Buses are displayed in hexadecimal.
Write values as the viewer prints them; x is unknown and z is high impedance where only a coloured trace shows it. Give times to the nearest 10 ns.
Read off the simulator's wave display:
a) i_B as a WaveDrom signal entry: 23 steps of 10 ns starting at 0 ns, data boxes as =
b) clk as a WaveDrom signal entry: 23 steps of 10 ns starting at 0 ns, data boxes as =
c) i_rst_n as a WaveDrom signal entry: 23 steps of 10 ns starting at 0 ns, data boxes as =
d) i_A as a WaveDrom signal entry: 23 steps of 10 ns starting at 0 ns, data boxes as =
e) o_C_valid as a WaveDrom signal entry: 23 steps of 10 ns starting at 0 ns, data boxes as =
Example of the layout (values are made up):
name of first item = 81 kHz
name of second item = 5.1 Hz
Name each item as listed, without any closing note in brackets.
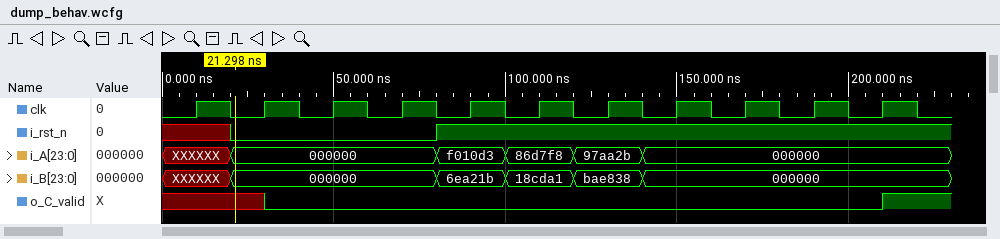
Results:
i_B as a WaveDrom signal entry: 23 steps of 10 ns starting at 0 ns, data boxes as = = {name: 'i_B', wave: 'x.=.....=.=.=.=........', data: '000000 6ea21b 18cda1 bae838 000000'}
clk as a WaveDrom signal entry: 23 steps of 10 ns starting at 0 ns, data boxes as = = {name: 'clk', wave: '01010101010101010101010'}
i_rst_n as a WaveDrom signal entry: 23 steps of 10 ns starting at 0 ns, data boxes as = = {name: 'i_rst_n', wave: 'x.0.....1..............'}
i_A as a WaveDrom signal entry: 23 steps of 10 ns starting at 0 ns, data boxes as = = {name: 'i_A', wave: 'x.=.....=.=.=.=........', data: '000000 f010d3 86d7f8 97aa2b 000000'}
o_C_valid as a WaveDrom signal entry: 23 steps of 10 ns starting at 0 ns, data boxes as = = {name: 'o_C_valid', wave: 'x..0.................1.'}
